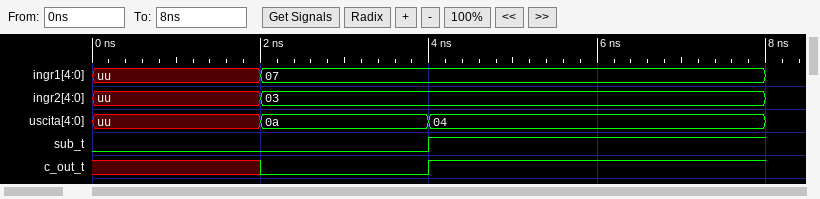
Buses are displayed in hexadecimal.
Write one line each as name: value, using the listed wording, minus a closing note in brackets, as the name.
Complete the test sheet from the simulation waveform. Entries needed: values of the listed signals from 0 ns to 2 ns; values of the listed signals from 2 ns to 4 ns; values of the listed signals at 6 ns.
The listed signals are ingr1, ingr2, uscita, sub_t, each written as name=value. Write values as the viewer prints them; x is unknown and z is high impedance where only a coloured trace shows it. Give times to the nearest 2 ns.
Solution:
values of the listed signals from 0 ns to 2 ns: ingr1=uu, ingr2=uu, uscita=uu, sub_t=0
values of the listed signals from 2 ns to 4 ns: ingr1=07, ingr2=03, uscita=0a, sub_t=0
values of the listed signals at 6 ns: ingr1=07, ingr2=03, uscita=04, sub_t=1
